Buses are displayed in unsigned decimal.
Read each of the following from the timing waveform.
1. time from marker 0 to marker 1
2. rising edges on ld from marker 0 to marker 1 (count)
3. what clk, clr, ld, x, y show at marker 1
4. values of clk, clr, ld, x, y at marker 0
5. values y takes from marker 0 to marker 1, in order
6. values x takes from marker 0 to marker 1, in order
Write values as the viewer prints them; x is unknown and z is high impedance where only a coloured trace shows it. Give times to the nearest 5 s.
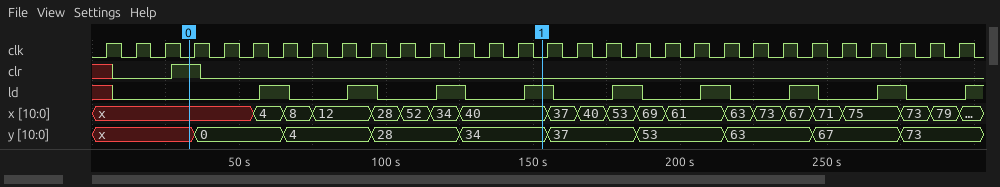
120 s
4
clk=0, clr=0, ld=1, x=40, y=34
clk=0, clr=1, ld=0, x=x, y=x
x, 0, 4, 28, 34
x, 4, 8, 12, 28, 52, 34, 40
